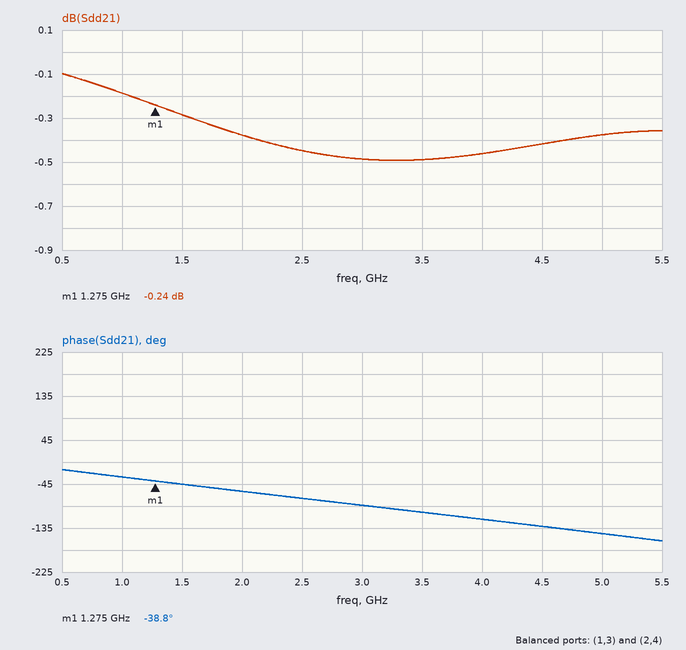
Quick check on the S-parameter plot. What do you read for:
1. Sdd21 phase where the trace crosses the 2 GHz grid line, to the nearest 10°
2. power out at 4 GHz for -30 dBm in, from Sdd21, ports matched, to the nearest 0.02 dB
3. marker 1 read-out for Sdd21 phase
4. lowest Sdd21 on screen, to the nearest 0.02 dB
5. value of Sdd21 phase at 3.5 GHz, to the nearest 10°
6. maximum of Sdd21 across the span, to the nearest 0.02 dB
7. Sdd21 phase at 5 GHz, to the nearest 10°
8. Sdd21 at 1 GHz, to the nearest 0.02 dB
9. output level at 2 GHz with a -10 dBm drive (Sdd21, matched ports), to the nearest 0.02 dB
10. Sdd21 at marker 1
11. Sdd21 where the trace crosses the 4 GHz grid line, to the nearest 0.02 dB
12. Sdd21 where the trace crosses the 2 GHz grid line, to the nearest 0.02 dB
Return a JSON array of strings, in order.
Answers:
["-60°", "-30.46 dBm", "-38.8°", "-0.50 dB", "-100°", "-0.10 dB", "-150°", "-0.18 dB", "-10.38 dBm", "-0.24 dB", "-0.46 dB", "-0.38 dB"]
